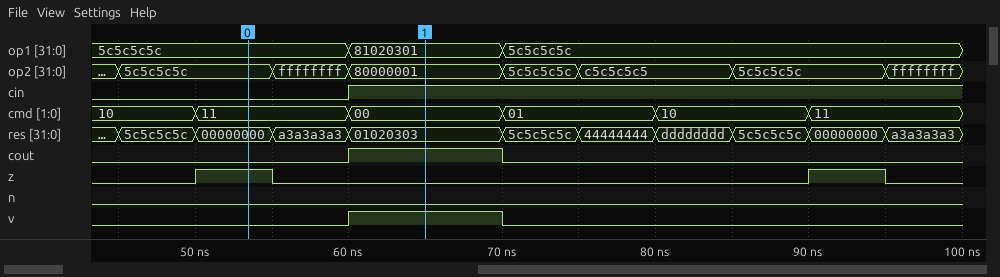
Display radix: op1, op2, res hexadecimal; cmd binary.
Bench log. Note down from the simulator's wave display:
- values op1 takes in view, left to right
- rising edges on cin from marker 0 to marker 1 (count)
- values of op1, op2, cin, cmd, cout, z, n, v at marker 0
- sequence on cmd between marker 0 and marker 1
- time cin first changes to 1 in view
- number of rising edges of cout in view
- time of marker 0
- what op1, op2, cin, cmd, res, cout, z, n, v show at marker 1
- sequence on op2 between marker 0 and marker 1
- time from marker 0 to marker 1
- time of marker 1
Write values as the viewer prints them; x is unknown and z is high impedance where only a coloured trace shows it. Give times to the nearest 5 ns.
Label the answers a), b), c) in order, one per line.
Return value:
a) 5c5c5c5c, 81020301, 5c5c5c5c
b) 1
c) op1=5c5c5c5c, op2=5c5c5c5c, cin=0, cmd=11, cout=0, z=1, n=0, v=0
d) 11, 00
e) 60 ns
f) 1
g) 55 ns
h) op1=81020301, op2=80000001, cin=1, cmd=00, res=01020303, cout=1, z=0, n=0, v=1
i) 5c5c5c5c, ffffffff, 80000001
j) 10 ns
k) 65 ns
